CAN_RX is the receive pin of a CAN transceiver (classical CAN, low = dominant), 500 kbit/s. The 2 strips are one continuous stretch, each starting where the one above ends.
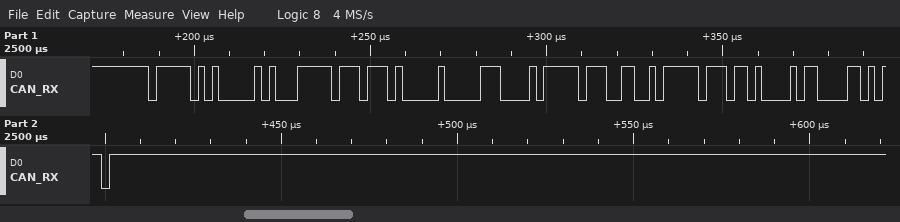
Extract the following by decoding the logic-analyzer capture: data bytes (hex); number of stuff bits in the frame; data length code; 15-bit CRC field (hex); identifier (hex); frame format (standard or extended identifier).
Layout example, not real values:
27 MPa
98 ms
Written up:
FF 74 00 C2 FF 32 FF 68
7
8
0x2C35
0x7E8
standard
